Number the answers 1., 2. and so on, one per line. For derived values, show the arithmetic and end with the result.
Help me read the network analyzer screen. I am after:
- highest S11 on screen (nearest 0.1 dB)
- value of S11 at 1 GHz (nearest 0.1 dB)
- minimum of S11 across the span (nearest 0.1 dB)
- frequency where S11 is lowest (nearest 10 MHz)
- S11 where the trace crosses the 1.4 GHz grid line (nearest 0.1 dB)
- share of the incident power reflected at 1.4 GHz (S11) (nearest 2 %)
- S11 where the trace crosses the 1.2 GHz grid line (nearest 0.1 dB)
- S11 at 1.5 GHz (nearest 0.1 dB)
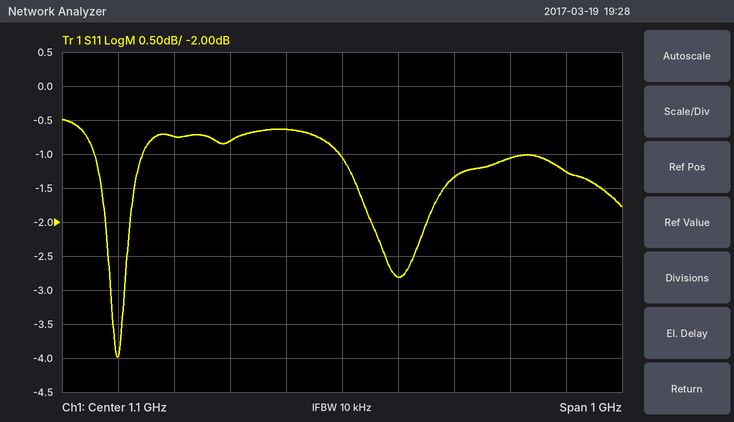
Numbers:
1. -0.5 dB
2. -0.6 dB
3. -4.0 dB
4. 700 MHz
5. -1.1 dB
6. 10^(-1.1/10) ≈ 78 %
7. -2.8 dB
8. -1.3 dB
